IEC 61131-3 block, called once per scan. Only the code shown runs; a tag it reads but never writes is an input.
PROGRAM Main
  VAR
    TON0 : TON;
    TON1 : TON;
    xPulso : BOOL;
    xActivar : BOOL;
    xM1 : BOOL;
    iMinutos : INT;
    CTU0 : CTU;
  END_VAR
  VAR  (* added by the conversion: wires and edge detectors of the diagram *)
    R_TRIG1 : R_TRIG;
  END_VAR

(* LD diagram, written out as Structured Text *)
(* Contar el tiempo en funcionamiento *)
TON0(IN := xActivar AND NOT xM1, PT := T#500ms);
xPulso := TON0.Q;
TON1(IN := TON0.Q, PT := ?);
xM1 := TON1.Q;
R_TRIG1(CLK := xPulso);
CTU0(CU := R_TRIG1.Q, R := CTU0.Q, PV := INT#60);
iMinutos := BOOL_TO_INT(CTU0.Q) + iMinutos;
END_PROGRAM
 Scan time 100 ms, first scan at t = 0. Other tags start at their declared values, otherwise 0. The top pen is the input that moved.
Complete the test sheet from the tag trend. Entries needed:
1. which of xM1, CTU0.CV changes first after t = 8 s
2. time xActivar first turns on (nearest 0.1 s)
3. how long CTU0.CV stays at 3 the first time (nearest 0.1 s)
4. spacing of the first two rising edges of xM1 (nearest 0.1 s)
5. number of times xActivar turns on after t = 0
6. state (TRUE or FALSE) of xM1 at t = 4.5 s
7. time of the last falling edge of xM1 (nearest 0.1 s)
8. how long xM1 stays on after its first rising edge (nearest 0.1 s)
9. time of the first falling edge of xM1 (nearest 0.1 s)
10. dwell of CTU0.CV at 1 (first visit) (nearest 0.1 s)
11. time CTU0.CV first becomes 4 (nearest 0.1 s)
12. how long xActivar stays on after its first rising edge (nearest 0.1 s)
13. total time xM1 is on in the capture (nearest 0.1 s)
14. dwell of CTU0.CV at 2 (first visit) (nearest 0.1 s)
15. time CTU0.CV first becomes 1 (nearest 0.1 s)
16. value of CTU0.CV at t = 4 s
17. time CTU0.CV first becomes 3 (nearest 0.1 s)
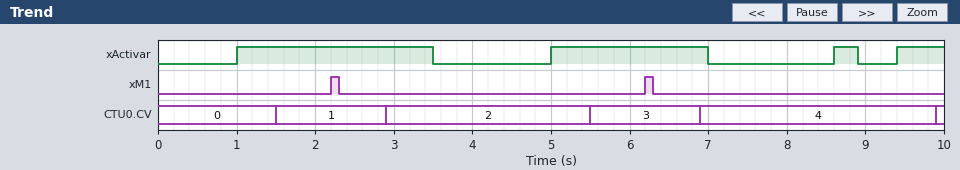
CTU0.CV
1.0 s
1.4 s
4.0 s
4
FALSE
6.3 s
0.1 s
2.3 s
1.4 s
6.9 s
2.5 s
0.2 s
2.6 s
1.5 s
2
5.5 s
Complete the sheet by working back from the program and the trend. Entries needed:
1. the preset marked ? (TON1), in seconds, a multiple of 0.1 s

0.7 s
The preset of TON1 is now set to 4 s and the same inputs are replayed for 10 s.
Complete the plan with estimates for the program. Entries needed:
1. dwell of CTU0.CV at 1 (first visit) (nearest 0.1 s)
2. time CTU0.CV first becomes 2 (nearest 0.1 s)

4.0 s
5.5 s
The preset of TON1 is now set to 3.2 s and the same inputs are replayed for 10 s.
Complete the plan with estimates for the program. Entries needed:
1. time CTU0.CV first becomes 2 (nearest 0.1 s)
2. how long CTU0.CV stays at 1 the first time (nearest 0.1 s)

5.5 s
4.0 s
